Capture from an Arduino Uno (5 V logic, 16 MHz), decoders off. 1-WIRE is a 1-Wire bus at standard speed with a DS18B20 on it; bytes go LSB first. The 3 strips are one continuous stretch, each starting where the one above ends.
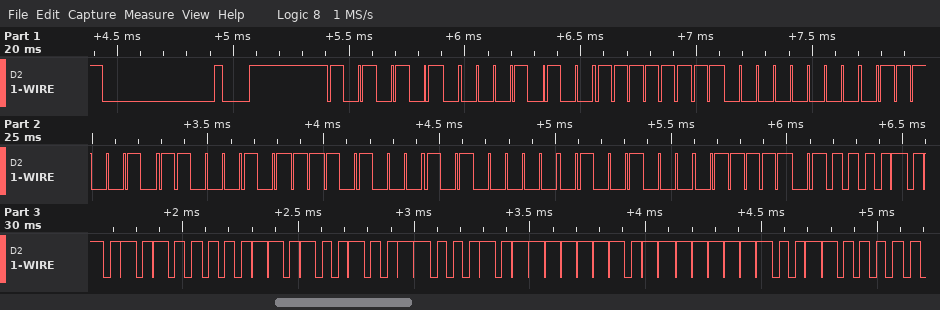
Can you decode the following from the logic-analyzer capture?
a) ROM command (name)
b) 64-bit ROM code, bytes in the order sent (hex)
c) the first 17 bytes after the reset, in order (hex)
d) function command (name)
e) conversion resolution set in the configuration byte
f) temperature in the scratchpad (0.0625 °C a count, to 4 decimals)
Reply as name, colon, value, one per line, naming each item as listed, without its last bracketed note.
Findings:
ROM command: Match ROM
64-bit ROM code, bytes in the order sent: 28 FF 00 4E A3 17 05 12
the first 17 bytes after the reset, in order: 55 28 FF 00 4E A3 17 05 12 BE 50 05 4B 46 7F FF 0C
function command: Read Scratchpad
conversion resolution set in the configuration byte: 12 bits
temperature in the scratchpad: 85.0000 °C
